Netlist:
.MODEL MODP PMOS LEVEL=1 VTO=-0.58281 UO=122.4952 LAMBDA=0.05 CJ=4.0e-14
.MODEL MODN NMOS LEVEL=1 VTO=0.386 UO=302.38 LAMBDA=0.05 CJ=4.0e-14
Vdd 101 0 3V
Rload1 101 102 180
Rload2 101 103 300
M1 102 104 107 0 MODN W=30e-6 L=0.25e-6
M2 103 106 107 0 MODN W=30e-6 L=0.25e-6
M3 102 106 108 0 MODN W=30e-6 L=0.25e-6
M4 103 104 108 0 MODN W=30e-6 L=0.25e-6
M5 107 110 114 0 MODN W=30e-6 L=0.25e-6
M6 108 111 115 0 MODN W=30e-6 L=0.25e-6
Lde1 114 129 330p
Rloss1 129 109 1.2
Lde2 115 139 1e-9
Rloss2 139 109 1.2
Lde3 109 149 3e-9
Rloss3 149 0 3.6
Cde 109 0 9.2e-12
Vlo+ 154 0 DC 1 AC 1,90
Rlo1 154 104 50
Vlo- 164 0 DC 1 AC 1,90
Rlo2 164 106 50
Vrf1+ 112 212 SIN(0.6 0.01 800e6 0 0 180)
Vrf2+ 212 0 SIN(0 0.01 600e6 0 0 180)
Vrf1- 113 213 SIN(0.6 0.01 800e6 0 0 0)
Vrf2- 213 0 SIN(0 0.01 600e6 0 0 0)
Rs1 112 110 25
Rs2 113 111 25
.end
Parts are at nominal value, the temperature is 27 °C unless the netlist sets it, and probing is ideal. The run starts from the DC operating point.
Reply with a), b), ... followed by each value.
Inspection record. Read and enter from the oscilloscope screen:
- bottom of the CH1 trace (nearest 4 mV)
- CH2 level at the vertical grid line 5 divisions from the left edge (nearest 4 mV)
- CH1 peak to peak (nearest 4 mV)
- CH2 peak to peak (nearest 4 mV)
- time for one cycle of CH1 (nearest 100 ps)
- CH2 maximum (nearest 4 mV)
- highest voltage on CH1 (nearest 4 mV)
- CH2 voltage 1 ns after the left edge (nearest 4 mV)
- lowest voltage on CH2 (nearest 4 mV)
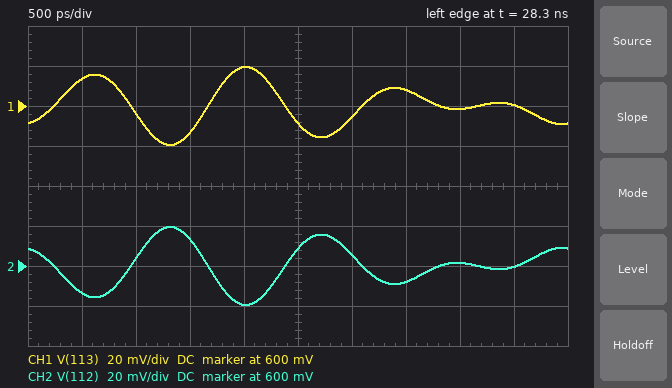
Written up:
a) 580 mV
b) 608 mV
c) 40 mV
d) 40 mV
e) 1.4 ns
f) 620 mV
g) 620 mV
h) 604 mV
i) 580 mV
